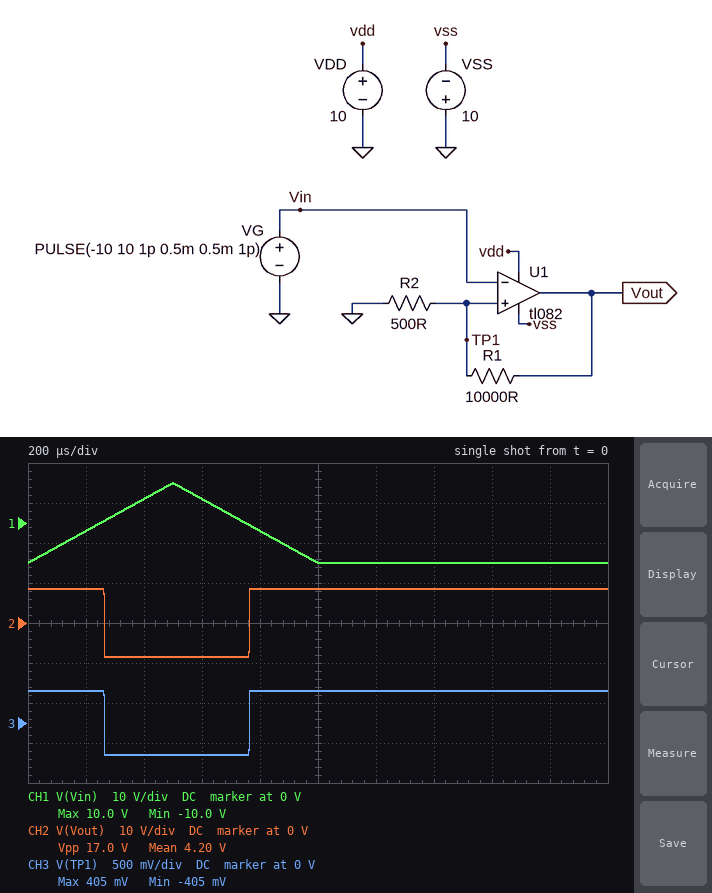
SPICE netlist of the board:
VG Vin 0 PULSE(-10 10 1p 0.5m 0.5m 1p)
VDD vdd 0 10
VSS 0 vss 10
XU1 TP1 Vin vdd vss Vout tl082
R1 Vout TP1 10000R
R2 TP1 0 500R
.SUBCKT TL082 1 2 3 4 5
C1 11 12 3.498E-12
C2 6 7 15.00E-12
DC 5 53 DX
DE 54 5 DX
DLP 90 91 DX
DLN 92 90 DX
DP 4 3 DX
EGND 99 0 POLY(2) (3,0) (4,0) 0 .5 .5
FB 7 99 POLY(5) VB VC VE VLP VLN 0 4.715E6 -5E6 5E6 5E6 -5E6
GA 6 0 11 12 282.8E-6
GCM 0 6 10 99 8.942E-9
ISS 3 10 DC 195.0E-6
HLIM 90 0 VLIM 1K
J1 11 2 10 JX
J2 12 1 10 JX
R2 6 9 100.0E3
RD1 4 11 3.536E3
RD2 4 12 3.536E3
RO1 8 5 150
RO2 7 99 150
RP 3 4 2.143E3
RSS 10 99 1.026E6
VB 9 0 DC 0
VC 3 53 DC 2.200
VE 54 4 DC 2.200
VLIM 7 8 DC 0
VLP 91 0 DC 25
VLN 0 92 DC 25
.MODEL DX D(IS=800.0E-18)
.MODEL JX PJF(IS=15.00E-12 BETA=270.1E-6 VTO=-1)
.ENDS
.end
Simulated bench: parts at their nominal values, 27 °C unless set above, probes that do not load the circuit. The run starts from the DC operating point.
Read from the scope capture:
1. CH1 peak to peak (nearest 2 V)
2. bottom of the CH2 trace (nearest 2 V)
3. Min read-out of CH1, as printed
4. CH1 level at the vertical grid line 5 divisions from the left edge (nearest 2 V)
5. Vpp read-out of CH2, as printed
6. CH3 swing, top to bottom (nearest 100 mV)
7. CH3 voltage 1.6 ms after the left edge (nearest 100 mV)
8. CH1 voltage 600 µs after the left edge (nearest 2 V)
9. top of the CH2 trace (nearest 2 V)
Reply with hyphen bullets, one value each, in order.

- 20 V
- -8 V
- -10.0 V
- -10 V
- 17.0 V
- 800 mV
- 400 mV
- 6 V
- 8 V
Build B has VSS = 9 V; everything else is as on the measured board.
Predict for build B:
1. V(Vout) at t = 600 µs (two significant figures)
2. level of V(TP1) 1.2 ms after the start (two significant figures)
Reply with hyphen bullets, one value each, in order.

- -7.5 V
- -360 mV
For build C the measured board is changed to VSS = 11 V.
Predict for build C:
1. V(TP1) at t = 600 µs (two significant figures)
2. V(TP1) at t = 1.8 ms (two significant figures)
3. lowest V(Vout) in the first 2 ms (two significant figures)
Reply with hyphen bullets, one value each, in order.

- -450 mV
- 400 mV
- -9.5 V
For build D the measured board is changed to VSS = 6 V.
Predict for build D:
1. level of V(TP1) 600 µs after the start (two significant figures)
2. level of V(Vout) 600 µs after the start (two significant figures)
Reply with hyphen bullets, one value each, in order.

- -210 mV
- -4.5 V
